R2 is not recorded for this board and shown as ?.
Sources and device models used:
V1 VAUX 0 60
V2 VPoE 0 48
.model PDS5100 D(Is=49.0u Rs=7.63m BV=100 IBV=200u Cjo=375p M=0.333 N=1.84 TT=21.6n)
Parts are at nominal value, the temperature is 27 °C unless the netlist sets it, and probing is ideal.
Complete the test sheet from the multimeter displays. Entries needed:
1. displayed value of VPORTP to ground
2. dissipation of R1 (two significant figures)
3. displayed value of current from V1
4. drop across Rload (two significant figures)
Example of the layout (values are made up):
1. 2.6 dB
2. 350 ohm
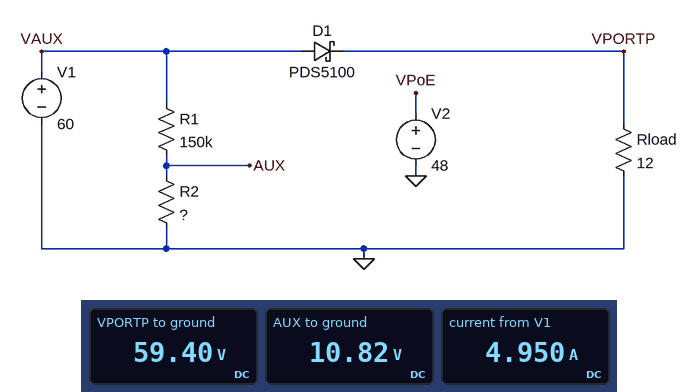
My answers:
1. 59.40 V
2. 16 mW
3. 4.950 A
4. 59 V
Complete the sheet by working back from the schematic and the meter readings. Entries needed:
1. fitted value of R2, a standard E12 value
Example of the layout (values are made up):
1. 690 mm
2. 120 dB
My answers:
1. 33 kΩ
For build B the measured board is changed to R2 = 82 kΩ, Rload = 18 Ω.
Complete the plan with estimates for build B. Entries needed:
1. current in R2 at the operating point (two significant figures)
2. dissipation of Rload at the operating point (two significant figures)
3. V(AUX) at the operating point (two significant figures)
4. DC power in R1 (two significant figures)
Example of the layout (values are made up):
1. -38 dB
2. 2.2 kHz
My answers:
1. 260 µA
2. 200 W
3. 21 V
4. 10 mW
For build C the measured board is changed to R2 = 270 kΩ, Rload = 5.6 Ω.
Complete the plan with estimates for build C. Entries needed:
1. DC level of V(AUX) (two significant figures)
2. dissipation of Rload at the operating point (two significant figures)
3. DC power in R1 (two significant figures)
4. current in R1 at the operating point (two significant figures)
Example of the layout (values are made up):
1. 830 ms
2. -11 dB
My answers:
1. 39 V
2. 630 W
3. 3.1 mW
4. 140 µA
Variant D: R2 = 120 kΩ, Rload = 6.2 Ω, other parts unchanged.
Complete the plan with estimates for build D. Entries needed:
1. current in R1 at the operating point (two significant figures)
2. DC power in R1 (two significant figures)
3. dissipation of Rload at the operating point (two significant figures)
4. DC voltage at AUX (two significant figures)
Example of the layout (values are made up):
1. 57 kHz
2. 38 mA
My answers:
1. 220 µA
2. 7.4 mW
3. 570 W
4. 27 V
